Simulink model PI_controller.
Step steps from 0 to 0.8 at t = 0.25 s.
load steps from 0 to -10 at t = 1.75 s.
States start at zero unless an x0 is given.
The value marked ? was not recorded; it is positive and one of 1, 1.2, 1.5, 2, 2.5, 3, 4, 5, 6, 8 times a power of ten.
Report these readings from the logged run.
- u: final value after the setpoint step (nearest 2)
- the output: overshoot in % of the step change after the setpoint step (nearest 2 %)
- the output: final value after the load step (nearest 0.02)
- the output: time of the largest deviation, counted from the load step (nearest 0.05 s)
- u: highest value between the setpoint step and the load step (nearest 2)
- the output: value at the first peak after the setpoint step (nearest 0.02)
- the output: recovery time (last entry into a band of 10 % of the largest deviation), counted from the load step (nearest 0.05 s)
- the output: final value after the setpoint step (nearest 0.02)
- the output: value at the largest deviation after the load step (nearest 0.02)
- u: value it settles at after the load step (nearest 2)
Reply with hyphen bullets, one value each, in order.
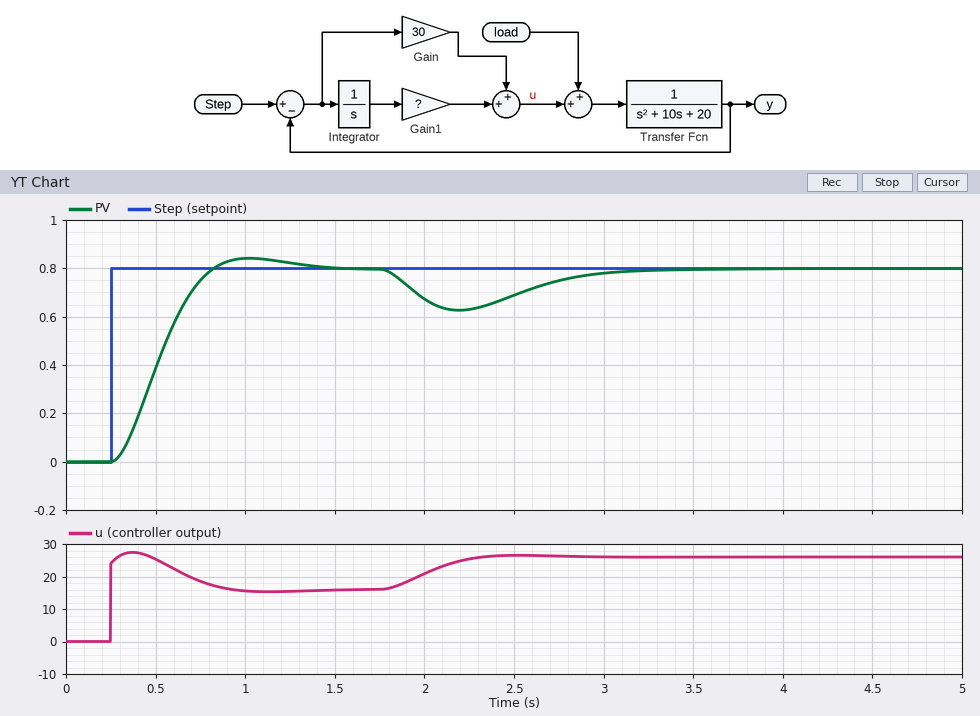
- 16
- 6 %
- 0.80
- 0.45 s
- 28
- 0.84
- 1.30 s
- 0.80
- 0.62
- 26
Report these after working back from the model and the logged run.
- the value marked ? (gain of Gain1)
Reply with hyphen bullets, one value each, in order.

- 80
